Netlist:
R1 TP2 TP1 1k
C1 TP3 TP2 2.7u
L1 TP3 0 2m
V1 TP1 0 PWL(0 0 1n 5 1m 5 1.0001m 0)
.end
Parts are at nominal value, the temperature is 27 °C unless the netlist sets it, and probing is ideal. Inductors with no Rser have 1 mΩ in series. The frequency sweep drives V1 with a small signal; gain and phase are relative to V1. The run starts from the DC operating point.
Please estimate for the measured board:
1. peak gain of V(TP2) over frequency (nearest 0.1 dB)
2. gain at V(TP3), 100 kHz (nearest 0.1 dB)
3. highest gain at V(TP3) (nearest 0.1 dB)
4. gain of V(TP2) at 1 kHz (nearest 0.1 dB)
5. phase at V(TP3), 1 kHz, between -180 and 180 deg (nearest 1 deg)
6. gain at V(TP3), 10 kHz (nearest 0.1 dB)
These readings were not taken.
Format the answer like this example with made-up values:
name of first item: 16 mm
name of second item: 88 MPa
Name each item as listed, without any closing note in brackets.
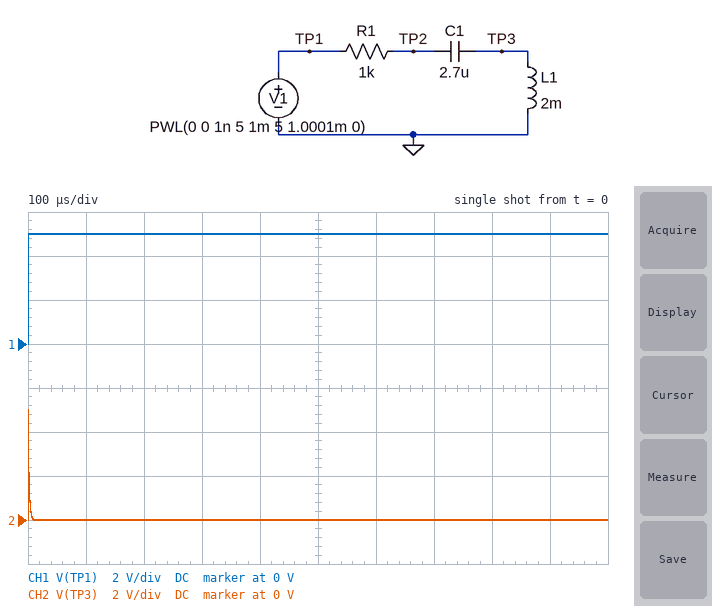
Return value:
peak gain of V(TP2) over frequency: 0 dB
gain at V(TP3), 100 kHz: -2.1 dB
highest gain at V(TP3): 0 dB
gain of V(TP2) at 1 kHz: -26.7 dB
phase at V(TP3), 1 kHz, between -180 and 180 deg: 93 deg
gain at V(TP3), 10 kHz: -18.1 dB
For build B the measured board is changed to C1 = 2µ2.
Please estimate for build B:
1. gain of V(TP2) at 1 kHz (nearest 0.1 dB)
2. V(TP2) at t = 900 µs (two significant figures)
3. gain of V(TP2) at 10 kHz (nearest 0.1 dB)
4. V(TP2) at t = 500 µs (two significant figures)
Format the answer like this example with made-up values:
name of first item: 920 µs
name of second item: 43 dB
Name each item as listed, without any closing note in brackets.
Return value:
gain of V(TP2) at 1 kHz: -24.5 dB
V(TP2) at t = 900 µs: 1.7 V
gain of V(TP2) at 10 kHz: -18.6 dB
V(TP2) at t = 500 µs: 1.0 V
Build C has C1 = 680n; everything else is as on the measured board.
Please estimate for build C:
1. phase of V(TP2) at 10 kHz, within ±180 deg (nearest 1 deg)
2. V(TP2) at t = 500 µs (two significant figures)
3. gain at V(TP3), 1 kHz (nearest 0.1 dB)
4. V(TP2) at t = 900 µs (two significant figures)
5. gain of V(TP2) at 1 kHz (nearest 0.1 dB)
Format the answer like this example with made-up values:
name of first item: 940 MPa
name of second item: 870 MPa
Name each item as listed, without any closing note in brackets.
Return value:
phase of V(TP2) at 10 kHz, within ±180 deg: 84 deg
V(TP2) at t = 500 µs: 2.6 V
gain at V(TP3), 1 kHz: -38.2 dB
V(TP2) at t = 900 µs: 3.7 V
gain of V(TP2) at 1 kHz: -13.3 dB
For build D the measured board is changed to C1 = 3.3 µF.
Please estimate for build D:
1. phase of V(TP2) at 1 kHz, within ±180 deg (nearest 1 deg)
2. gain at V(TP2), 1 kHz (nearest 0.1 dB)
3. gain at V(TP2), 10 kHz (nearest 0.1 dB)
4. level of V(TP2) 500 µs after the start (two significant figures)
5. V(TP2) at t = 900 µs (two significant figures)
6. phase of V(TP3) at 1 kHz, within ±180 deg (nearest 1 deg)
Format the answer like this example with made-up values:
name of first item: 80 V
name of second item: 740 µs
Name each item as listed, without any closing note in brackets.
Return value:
phase of V(TP2) at 1 kHz, within ±180 deg: -88 deg
gain at V(TP2), 1 kHz: -29.0 dB
gain at V(TP2), 10 kHz: -18.4 dB
level of V(TP2) 500 µs after the start: 700 mV
V(TP2) at t = 900 µs: 1.2 V
phase of V(TP3) at 1 kHz, within ±180 deg: 92 deg
